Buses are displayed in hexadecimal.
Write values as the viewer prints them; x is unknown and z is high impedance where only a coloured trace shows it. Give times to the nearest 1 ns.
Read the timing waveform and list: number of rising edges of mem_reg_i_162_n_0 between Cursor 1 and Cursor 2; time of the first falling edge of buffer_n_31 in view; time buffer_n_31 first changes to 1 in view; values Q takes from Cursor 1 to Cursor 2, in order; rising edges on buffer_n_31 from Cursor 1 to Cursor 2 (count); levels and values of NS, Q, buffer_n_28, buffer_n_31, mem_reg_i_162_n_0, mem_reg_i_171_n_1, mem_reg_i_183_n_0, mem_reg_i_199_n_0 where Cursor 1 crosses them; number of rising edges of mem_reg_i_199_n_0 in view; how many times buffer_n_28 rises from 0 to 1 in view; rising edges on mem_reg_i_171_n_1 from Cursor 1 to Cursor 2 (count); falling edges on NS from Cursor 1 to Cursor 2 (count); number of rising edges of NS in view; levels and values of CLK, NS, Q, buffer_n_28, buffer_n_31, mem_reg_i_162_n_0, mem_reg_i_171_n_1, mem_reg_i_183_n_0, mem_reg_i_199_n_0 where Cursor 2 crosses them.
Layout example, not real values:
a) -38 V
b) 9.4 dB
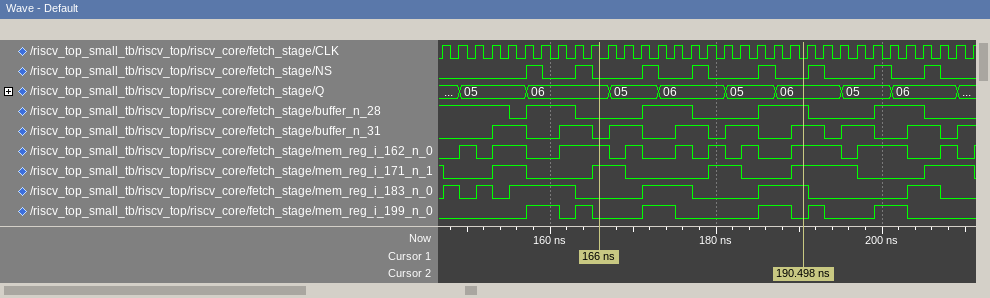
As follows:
a) 5
b) 157 ns
c) 153 ns
d) 06, 05, 06, 05, 06
e) 4
f) NS=0, Q=06, buffer_n_28=0, buffer_n_31=0, mem_reg_i_162_n_0=1, mem_reg_i_171_n_1=1, mem_reg_i_183_n_0=0, mem_reg_i_199_n_0=0
g) 6
h) 4
i) 2
j) 3
k) 8
l) CLK=0, NS=0, Q=06, buffer_n_28=1, buffer_n_31=1, mem_reg_i_162_n_0=1, mem_reg_i_171_n_1=1, mem_reg_i_183_n_0=1, mem_reg_i_199_n_0=0
